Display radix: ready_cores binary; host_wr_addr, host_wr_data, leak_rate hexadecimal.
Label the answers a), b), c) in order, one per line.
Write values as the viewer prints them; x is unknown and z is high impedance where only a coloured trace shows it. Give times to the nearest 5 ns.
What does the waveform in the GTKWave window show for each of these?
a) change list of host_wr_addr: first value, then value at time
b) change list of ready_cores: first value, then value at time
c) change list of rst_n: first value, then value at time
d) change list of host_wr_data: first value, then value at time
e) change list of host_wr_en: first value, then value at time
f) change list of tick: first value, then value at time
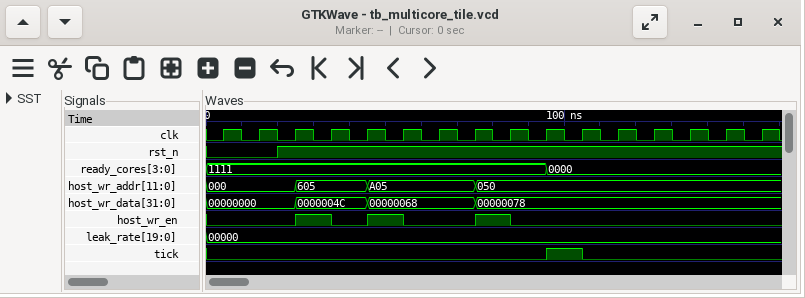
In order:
a) 000, 605 at 25 ns, A05 at 45 ns, 050 at 75 ns
b) 1111, 0000 at 95 ns
c) 0, 1 at 20 ns
d) 00000000, 0000004C at 25 ns, 00000068 at 45 ns, 00000078 at 75 ns
e) 0, 1 at 25 ns, 0 at 35 ns, 1 at 45 ns, 0 at 55 ns, 1 at 75 ns, 0 at 85 ns
f) 0, 1 at 95 ns, 0 at 105 ns
